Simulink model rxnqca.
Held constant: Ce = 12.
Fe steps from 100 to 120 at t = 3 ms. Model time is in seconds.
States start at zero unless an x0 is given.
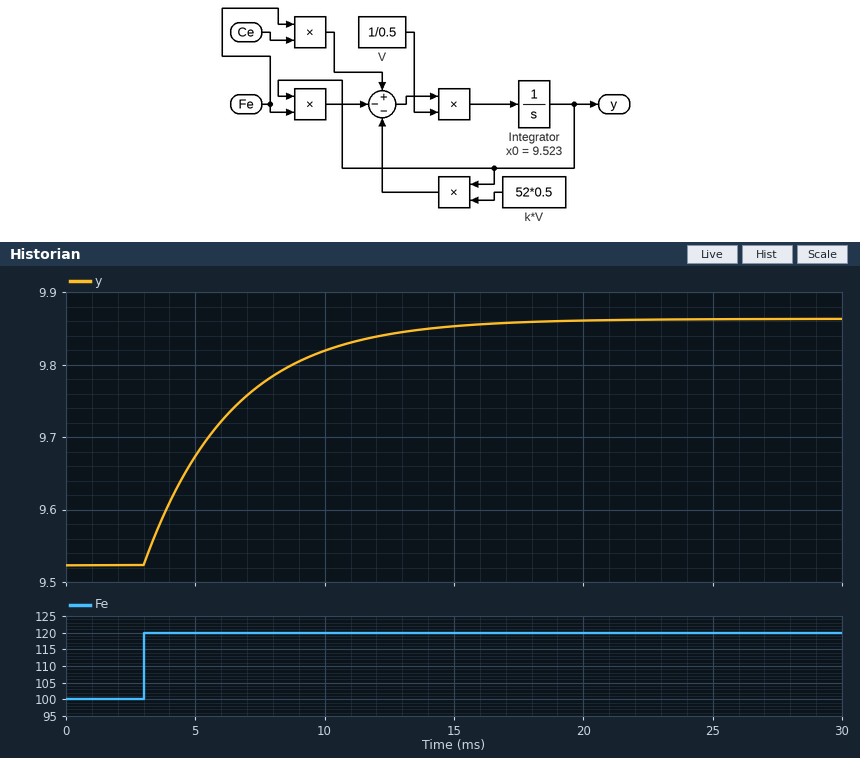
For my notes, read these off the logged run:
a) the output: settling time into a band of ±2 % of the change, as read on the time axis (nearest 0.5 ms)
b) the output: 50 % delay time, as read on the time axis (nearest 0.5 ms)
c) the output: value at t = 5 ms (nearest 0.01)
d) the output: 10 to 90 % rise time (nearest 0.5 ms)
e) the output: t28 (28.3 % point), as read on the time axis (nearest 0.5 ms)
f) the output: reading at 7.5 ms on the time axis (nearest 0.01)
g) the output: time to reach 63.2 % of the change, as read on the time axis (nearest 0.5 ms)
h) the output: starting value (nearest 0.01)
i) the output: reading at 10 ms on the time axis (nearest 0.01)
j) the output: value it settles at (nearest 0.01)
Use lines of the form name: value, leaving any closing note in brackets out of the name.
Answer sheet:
the output: settling time into a band of ±2 % of the change, as read on the time axis: 16.5 ms
the output: 50 % delay time, as read on the time axis: 5.5 ms
the output: value at t = 5 ms: 9.67
the output: 10 to 90 % rise time: 7.5 ms
the output: t28 (28.3 % point), as read on the time axis: 4.0 ms
the output: reading at 7.5 ms on the time axis: 9.77
the output: time to reach 63.2 % of the change, as read on the time axis: 6.5 ms
the output: starting value: 9.52
the output: reading at 10 ms on the time axis: 9.82
the output: value it settles at: 9.86
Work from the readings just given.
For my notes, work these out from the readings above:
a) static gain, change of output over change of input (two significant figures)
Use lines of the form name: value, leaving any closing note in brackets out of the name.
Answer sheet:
static gain, change of output over change of input: 0.017
